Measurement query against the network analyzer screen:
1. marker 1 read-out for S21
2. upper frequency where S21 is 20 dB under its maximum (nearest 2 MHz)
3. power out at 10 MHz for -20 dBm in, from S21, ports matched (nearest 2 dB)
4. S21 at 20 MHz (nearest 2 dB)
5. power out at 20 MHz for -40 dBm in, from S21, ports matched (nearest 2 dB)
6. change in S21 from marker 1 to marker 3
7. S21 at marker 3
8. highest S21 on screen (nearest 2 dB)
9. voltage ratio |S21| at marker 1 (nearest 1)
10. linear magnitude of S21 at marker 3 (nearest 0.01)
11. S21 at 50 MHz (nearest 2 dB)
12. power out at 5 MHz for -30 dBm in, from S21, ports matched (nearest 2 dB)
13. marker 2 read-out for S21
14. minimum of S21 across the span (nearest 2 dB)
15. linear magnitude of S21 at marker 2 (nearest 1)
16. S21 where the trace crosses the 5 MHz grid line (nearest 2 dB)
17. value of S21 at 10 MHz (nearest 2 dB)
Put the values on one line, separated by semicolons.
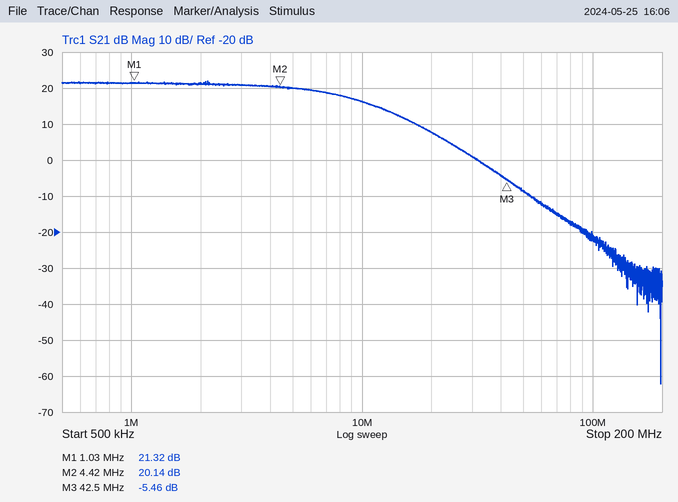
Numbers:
21.32 dB; 28 MHz; -4 dBm; 8 dB; -32 dBm; -26.78 dB; -5.46 dB; 22 dB; 12; 0.53; -8 dB; -10 dBm; 20.14 dB; -62 dB; 10; 20 dB; 16 dB
